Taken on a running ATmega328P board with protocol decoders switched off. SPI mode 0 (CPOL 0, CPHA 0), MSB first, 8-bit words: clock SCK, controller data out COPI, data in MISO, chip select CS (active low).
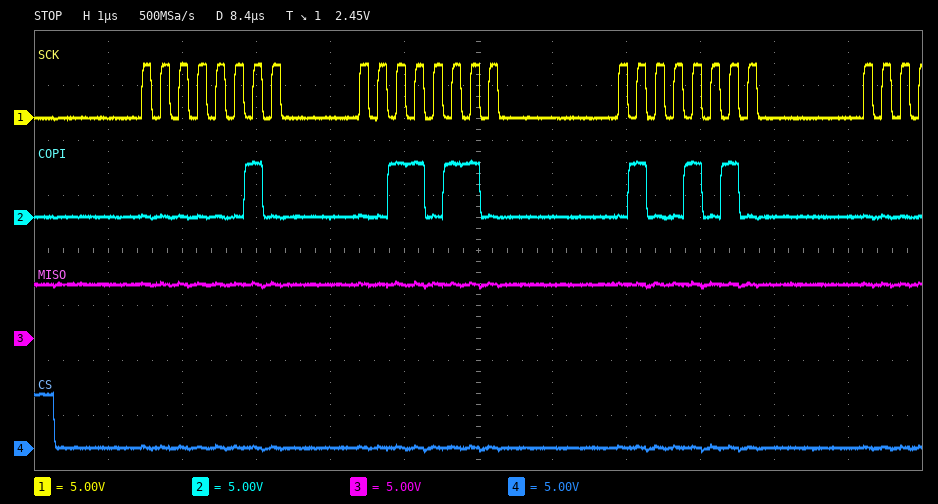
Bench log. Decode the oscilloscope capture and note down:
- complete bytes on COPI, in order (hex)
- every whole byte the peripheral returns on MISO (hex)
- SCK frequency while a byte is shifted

02 36 4A
FF FF FF
4 MHz
